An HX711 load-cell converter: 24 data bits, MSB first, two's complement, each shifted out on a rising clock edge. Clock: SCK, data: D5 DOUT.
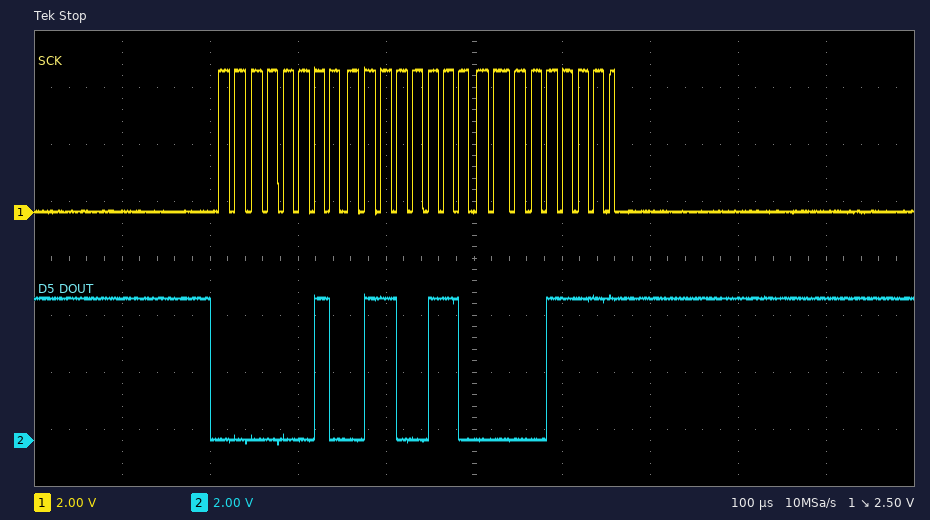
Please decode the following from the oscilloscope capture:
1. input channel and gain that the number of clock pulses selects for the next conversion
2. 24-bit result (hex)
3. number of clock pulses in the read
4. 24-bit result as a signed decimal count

channel A, gain 128
0x02660F
25
157199
